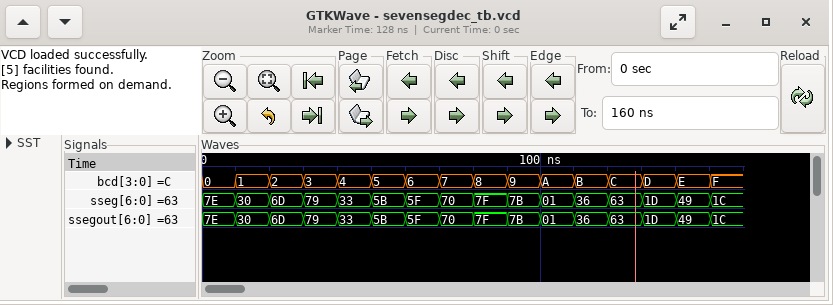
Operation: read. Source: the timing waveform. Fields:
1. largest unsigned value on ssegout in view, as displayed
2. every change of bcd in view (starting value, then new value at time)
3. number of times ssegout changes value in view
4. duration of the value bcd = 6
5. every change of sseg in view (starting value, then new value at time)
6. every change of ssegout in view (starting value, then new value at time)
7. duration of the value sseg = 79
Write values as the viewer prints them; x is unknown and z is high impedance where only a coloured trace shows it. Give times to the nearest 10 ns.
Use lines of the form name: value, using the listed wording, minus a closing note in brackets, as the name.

largest unsigned value on ssegout in view, as displayed: 7F
every change of bcd in view: 0, 1 at 10 ns, 2 at 20 ns, 3 at 30 ns, 4 at 40 ns, 5 at 50 ns, 6 at 60 ns, 7 at 70 ns, 8 at 80 ns, 9 at 90 ns, A at 100 ns, B at 110 ns, C at 120 ns, D at 130 ns, E at 140 ns, F at 150 ns
number of times ssegout changes value in view: 15
duration of the value bcd = 6: 10 ns
every change of sseg in view: 7E, 30 at 10 ns, 6D at 20 ns, 79 at 30 ns, 33 at 40 ns, 5B at 50 ns, 5F at 60 ns, 70 at 70 ns, 7F at 80 ns, 7B at 90 ns, 01 at 100 ns, 36 at 110 ns, 63 at 120 ns, 1D at 130 ns, 49 at 140 ns, 1C at 150 ns
every change of ssegout in view: 7E, 30 at 10 ns, 6D at 20 ns, 79 at 30 ns, 33 at 40 ns, 5B at 50 ns, 5F at 60 ns, 70 at 70 ns, 7F at 80 ns, 7B at 90 ns, 01 at 100 ns, 36 at 110 ns, 63 at 120 ns, 1D at 130 ns, 49 at 140 ns, 1C at 150 ns
duration of the value sseg = 79: 10 ns
